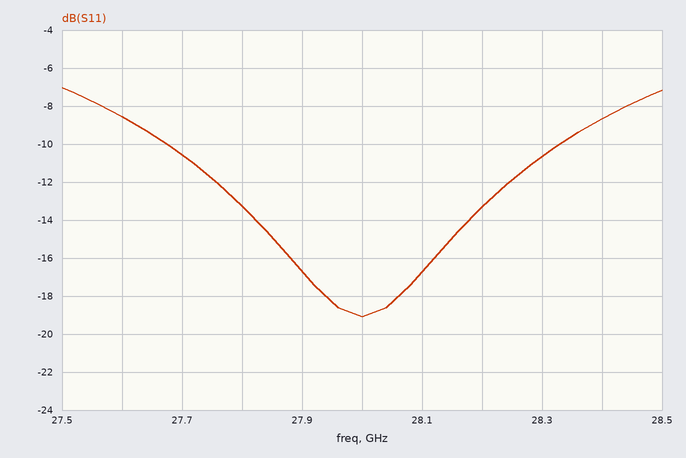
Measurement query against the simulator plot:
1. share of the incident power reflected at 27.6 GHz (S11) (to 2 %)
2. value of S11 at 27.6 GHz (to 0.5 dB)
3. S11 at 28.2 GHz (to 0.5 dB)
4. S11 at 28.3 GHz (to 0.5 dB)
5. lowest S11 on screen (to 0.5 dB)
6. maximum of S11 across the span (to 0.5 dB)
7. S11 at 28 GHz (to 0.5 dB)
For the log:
14 %
-8.5 dB
-13.5 dB
-10.5 dB
-19.0 dB
-7.0 dB
-19.0 dB
